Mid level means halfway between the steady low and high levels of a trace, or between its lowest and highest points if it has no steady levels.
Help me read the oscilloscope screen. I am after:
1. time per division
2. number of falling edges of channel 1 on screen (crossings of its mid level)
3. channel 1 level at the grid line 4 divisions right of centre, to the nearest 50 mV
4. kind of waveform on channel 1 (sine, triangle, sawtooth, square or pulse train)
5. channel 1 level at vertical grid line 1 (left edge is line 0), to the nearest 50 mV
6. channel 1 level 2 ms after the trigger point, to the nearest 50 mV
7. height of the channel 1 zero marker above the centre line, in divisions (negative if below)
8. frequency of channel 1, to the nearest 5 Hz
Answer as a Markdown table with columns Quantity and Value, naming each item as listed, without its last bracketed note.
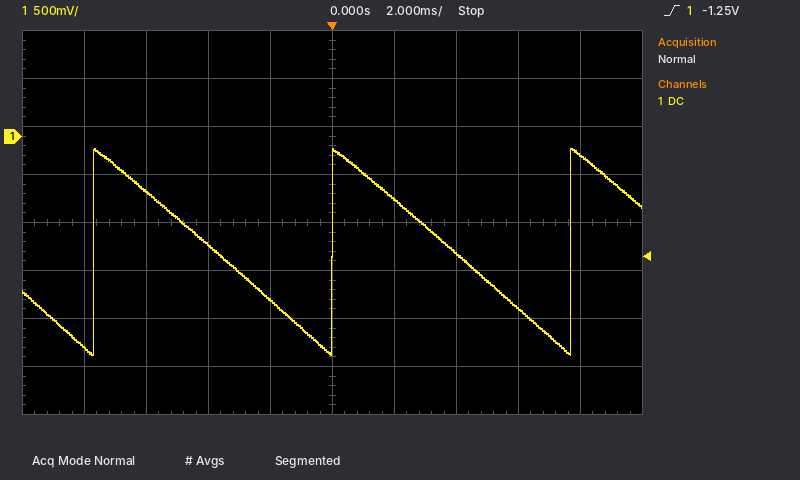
| Quantity | Value |
|---|---|
| time per division | 2 ms |
| number of falling edges of channel 1 on screen | 2 |
| channel 1 level at the grid line 4 divisions right of centre, to the nearest 50 mV | -200 mV |
| kind of waveform on channel 1 | sawtooth |
| channel 1 level at vertical grid line 1 (left edge is line 0), to the nearest 50 mV | -2.20 V |
| channel 1 level 2 ms after the trigger point, to the nearest 50 mV | -650 mV |
| height of the channel 1 zero marker above the centre line, in divisions | +1.8 div |
| frequency of channel 1, to the nearest 5 Hz | 130 Hz |
